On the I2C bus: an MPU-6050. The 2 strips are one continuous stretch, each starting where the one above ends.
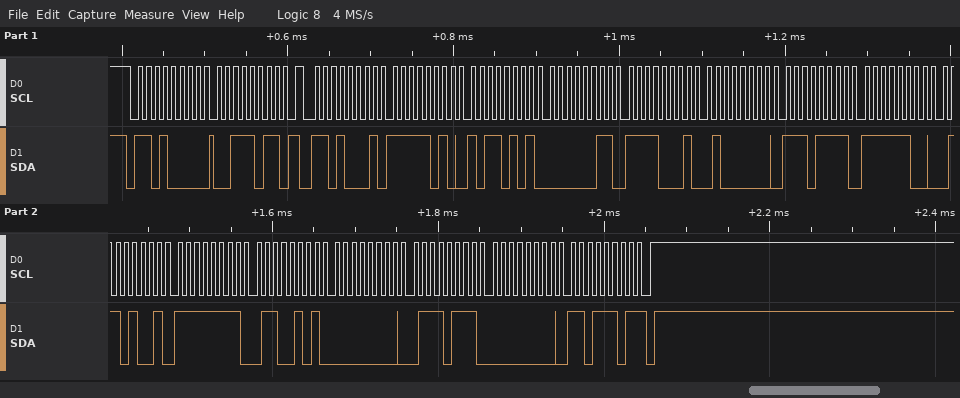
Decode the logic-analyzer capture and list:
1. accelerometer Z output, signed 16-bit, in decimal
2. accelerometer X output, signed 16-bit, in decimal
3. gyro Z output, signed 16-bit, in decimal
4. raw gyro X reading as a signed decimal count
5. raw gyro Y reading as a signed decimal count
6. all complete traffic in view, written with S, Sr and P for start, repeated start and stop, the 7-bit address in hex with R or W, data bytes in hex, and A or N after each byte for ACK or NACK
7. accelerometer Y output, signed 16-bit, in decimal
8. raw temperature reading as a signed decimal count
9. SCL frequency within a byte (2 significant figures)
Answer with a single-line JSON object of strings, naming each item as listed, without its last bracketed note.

{"accelerometer Z output, signed 16-bit, in decimal": "16623", "accelerometer X output, signed 16-bit, in decimal": "-1355", "gyro Z output, signed 16-bit, in decimal": "221", "raw gyro X reading as a signed decimal count": "-155", "raw gyro Y reading as a signed decimal count": "119", "all complete traffic in view, written with S, Sr and P for start, repeated start and stop, the 7-bit address in hex with R or W, data bytes in hex, and A or N after each byte for ACK or NACK": "S 68W A 3B A Sr 68R A FA A B5 A 03 A F1 A 40 A EF A FC A 69 A FF A 65 A 00 A 77 A 00 A DD N P", "accelerometer Y output, signed 16-bit, in decimal": "1009", "raw temperature reading as a signed decimal count": "-919", "SCL frequency within a byte": "100 kHz"}
